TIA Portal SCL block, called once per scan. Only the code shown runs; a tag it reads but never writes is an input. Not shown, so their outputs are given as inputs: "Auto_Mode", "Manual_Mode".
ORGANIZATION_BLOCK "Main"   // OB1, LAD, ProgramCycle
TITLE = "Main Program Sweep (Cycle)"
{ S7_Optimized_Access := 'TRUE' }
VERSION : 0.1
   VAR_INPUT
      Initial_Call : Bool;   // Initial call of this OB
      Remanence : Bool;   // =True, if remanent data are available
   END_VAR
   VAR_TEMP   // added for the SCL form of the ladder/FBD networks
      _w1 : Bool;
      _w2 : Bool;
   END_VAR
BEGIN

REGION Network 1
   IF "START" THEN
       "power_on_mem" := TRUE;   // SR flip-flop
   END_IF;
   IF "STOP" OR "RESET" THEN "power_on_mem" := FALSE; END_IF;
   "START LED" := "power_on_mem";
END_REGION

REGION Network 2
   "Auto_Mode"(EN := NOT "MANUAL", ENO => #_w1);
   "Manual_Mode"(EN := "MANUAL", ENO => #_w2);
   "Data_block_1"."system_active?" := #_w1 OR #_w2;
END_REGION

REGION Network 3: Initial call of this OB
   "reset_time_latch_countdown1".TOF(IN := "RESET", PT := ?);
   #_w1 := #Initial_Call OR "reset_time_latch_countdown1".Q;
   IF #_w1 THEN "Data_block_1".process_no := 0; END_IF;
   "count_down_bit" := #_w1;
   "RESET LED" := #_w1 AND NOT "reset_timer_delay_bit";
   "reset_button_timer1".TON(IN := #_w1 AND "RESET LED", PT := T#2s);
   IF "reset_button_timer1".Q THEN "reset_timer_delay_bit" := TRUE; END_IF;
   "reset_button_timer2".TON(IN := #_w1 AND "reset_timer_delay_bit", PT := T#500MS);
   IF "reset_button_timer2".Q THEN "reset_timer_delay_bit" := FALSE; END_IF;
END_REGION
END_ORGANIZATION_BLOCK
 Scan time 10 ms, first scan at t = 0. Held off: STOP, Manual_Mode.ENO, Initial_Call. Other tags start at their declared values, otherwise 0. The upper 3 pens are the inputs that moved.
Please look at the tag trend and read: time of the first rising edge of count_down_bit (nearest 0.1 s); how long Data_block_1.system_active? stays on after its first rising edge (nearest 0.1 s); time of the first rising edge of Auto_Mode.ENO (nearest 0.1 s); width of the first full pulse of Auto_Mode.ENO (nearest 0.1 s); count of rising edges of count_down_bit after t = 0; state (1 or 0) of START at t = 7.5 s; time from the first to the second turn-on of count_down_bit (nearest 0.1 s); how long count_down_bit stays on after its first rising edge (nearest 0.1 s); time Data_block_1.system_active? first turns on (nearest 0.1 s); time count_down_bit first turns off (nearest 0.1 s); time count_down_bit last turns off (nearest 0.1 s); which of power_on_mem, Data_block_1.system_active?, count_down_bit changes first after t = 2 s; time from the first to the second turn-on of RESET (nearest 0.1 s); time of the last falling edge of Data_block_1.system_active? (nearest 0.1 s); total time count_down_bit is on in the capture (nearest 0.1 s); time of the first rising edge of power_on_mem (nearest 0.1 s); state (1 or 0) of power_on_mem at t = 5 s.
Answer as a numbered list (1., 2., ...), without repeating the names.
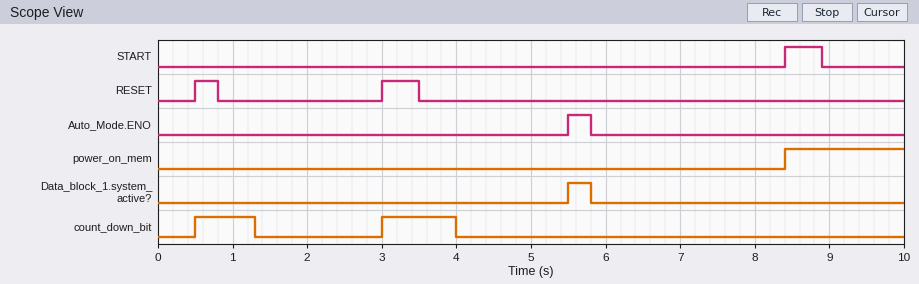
1. 0.5 s
2. 0.3 s
3. 5.5 s
4. 0.3 s
5. 2
6. 0
7. 2.5 s
8. 0.8 s
9. 5.5 s
10. 1.3 s
11. 4.0 s
12. count_down_bit
13. 2.5 s
14. 5.8 s
15. 1.8 s
16. 8.4 s
17. 0
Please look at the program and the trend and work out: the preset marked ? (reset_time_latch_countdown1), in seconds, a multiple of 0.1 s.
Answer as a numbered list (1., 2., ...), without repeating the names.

1. 0.5 s
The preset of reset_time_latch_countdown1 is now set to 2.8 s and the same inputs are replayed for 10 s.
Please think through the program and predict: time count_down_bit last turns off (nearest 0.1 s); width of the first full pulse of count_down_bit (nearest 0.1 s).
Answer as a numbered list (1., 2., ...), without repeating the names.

1. 6.3 s
2. 5.8 s
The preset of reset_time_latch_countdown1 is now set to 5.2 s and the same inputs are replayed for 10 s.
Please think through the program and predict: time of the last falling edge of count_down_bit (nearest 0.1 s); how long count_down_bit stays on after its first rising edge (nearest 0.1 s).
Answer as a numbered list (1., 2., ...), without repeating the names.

1. 8.7 s
2. 8.2 s
